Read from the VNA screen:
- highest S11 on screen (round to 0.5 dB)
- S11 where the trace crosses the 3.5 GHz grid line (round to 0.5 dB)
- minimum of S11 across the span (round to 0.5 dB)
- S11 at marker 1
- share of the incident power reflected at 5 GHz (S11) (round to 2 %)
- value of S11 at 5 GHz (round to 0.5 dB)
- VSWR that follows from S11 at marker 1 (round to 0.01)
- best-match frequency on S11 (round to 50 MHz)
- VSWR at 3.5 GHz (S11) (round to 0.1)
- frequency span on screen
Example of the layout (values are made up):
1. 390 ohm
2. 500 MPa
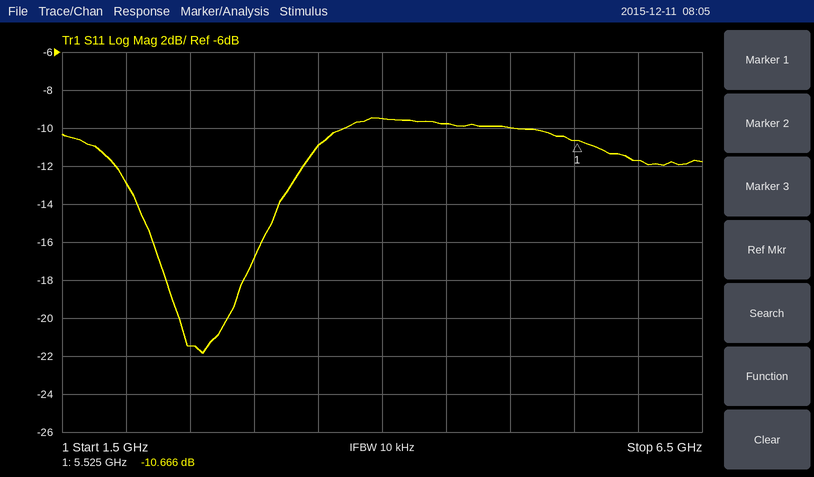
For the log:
1. -9.5 dB
2. -11.0 dB
3. -22.0 dB
4. -10.666 dB
5. 10 %
6. -10.0 dB
7. 1.83
8. 2.60 GHz
9. 1.8
10. 5 GHz
